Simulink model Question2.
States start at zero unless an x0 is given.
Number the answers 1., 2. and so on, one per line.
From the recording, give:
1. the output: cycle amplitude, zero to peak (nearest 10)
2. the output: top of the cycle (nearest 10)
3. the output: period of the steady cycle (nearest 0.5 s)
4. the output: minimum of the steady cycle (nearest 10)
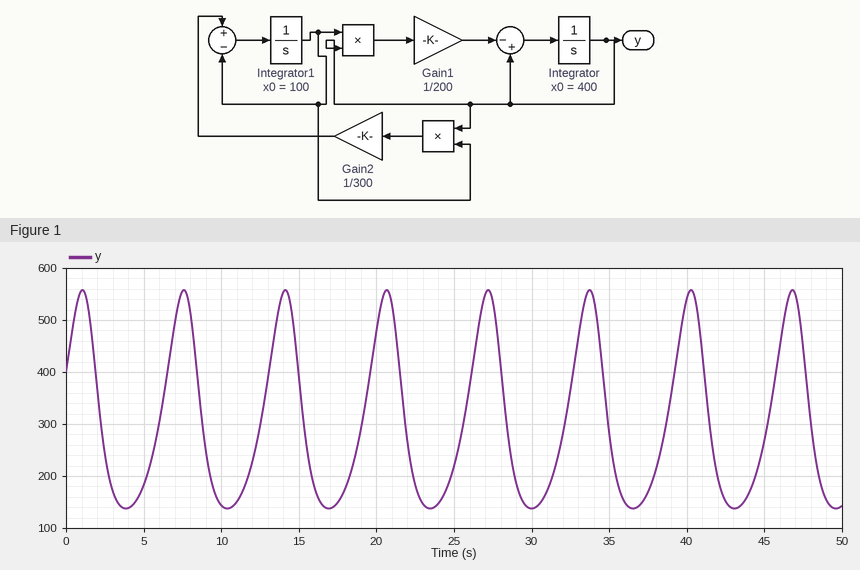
1. 210
2. 560
3. 6.5 s
4. 140
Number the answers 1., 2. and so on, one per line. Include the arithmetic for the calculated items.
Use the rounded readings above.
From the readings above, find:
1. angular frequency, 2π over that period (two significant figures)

1. 2π / 6.5 = 0.97 rad/s
